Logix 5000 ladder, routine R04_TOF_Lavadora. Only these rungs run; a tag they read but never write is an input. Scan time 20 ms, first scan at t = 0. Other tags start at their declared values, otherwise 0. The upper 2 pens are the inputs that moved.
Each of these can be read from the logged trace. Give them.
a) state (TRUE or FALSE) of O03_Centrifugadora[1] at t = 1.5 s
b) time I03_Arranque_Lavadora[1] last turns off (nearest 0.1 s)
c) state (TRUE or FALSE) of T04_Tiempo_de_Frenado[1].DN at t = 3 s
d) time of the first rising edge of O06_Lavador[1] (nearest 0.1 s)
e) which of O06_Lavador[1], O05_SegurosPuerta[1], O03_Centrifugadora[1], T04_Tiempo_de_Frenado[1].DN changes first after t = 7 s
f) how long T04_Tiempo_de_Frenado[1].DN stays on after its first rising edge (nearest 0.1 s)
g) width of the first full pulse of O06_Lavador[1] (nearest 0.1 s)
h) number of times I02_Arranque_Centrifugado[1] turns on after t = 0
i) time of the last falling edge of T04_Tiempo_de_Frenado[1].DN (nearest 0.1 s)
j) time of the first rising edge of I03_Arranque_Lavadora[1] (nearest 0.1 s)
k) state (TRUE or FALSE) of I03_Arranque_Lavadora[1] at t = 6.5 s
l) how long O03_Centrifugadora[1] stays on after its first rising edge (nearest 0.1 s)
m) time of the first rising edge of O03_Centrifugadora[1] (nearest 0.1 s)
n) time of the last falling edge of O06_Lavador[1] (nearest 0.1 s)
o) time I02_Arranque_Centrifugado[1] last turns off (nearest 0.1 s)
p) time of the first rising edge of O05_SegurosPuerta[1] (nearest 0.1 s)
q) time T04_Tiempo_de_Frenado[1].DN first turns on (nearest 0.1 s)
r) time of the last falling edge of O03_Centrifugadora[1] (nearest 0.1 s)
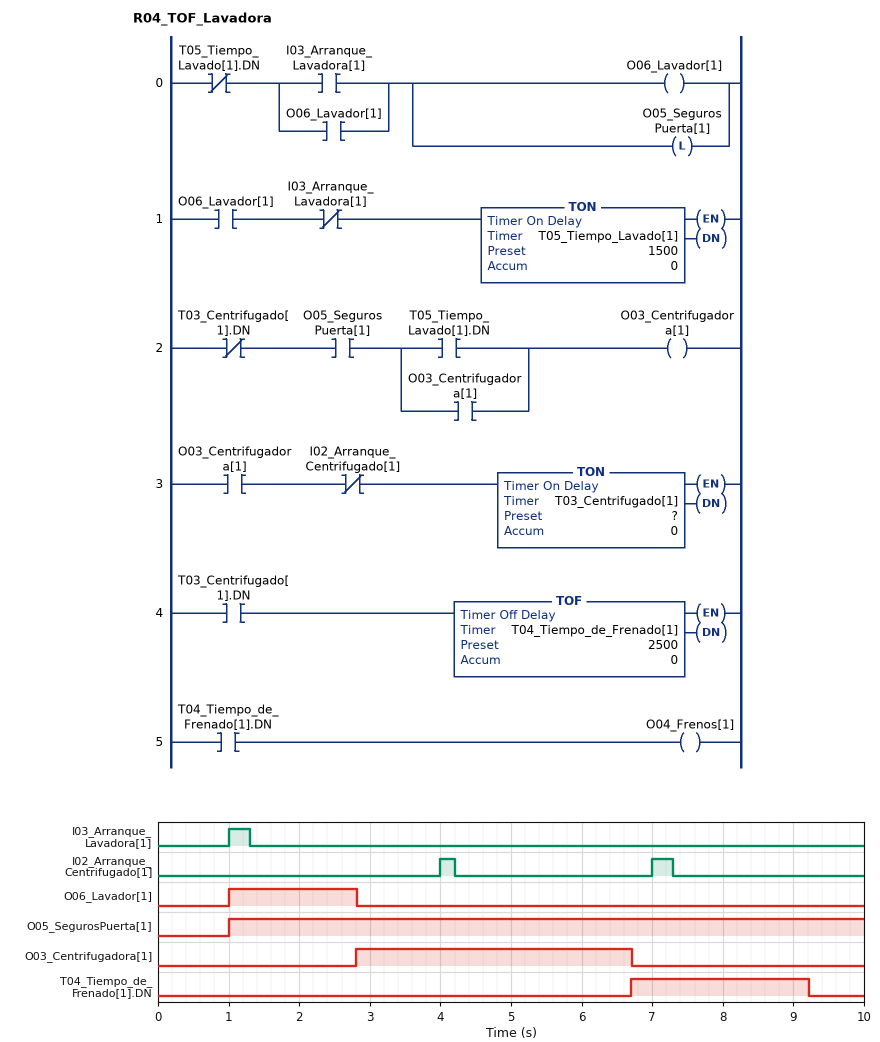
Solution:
FALSE
1.3 s
FALSE
1.0 s
T04_Tiempo_de_Frenado[1].DN
2.5 s
1.8 s
2
9.2 s
1.0 s
FALSE
3.9 s
2.8 s
2.8 s
7.3 s
1.0 s
6.7 s
6.7 s
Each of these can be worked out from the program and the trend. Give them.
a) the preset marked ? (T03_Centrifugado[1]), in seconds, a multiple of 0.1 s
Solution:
2.5 s
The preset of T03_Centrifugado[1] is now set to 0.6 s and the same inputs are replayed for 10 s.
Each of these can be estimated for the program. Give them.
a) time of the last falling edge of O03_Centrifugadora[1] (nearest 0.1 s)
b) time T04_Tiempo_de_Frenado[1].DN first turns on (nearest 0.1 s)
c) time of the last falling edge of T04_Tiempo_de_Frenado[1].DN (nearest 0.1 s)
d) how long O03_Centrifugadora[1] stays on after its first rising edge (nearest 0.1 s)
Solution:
3.4 s
3.4 s
5.9 s
0.6 s
